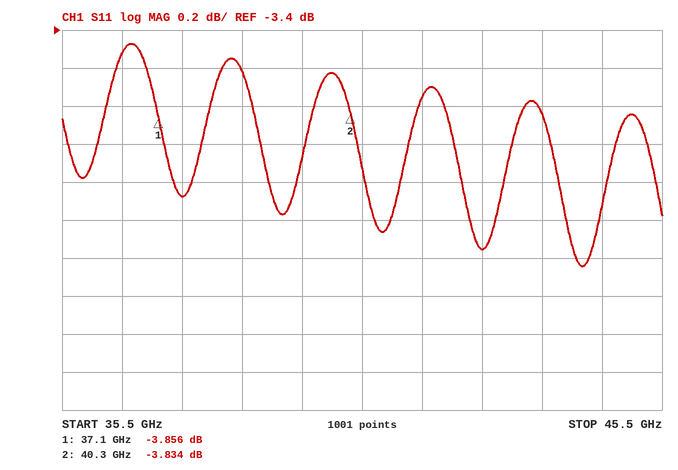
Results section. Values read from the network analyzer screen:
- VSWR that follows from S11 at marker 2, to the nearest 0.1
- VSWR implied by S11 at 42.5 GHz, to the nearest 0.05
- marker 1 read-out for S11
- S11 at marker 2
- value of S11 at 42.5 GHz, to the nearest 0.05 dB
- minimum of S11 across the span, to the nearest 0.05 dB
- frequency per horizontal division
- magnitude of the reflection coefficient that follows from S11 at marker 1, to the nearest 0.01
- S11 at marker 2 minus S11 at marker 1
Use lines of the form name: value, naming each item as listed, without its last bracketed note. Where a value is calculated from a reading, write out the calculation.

VSWR that follows from S11 at marker 2, to the nearest 0.1: (1 + 0.6431)/(1 − 0.6431) ≈ 4.6
VSWR implied by S11 at 42.5 GHz, to the nearest 0.05: |Γ| = 10^(-4.55/20) = 0.5922; VSWR = (1 + 0.5922)/(1 − 0.5922) ≈ 3.90
marker 1 read-out for S11: -3.856 dB
S11 at marker 2: -3.834 dB
value of S11 at 42.5 GHz, to the nearest 0.05 dB: -4.55 dB
minimum of S11 across the span, to the nearest 0.05 dB: -4.65 dB
frequency per horizontal division: 1 GHz
magnitude of the reflection coefficient that follows from S11 at marker 1, to the nearest 0.01: 10^(-3.856/20) ≈ 0.64
S11 at marker 2 minus S11 at marker 1: -3.834 − (-3.856) = 0.022 dB
